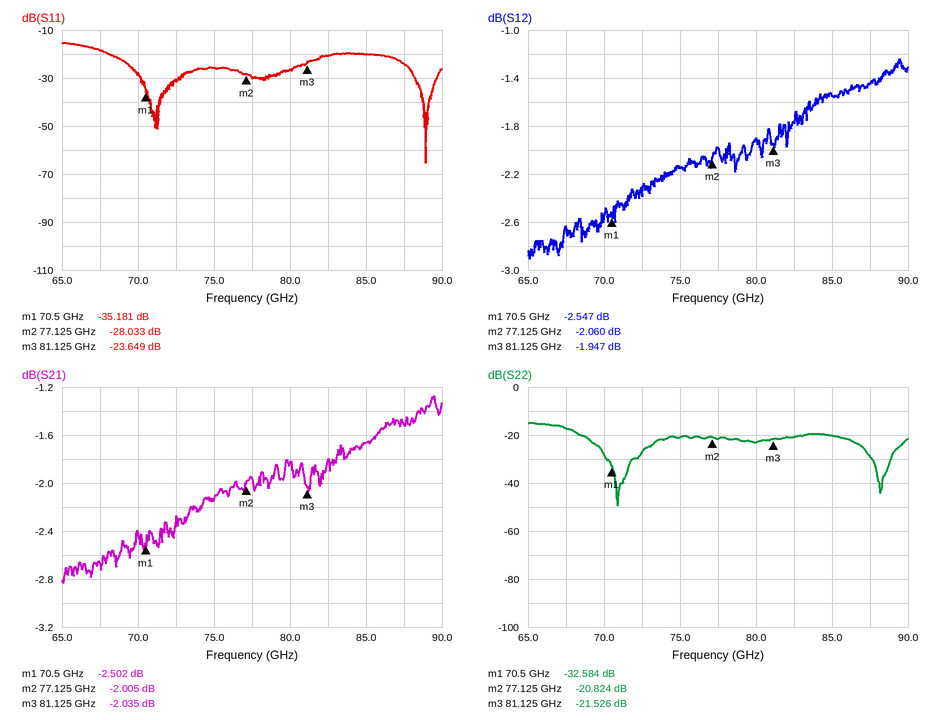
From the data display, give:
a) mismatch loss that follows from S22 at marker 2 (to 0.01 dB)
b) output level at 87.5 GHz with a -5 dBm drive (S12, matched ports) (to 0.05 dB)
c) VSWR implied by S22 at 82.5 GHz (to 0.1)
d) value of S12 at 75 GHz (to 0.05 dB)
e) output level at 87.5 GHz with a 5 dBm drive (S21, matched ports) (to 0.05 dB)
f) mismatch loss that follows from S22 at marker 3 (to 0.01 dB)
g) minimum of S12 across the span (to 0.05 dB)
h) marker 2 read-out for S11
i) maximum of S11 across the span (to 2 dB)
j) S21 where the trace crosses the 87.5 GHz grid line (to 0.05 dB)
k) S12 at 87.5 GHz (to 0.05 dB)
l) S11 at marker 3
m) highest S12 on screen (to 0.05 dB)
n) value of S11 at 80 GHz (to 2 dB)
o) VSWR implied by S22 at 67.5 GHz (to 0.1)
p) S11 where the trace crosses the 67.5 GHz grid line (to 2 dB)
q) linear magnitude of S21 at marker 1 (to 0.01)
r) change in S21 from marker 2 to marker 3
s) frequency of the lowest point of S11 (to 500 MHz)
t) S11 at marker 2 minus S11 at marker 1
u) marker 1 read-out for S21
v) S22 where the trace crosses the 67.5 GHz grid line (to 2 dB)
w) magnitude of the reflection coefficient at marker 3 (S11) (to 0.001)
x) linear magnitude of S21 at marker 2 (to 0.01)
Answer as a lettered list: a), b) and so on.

a) 0.04 dB
b) -6.45 dBm
c) 1.2
d) -2.15 dB
e) 3.50 dBm
f) 0.03 dB
g) -2.90 dB
h) -28.033 dB
i) -16 dB
j) -1.50 dB
k) -1.45 dB
l) -23.649 dB
m) -1.25 dB
n) -26 dB
o) 1.3
p) -18 dB
q) 0.75
r) -0.030 dB
s) 89.0 GHz
t) 7.148 dB
u) -2.502 dB
v) -18 dB
w) 0.066
x) 0.79
